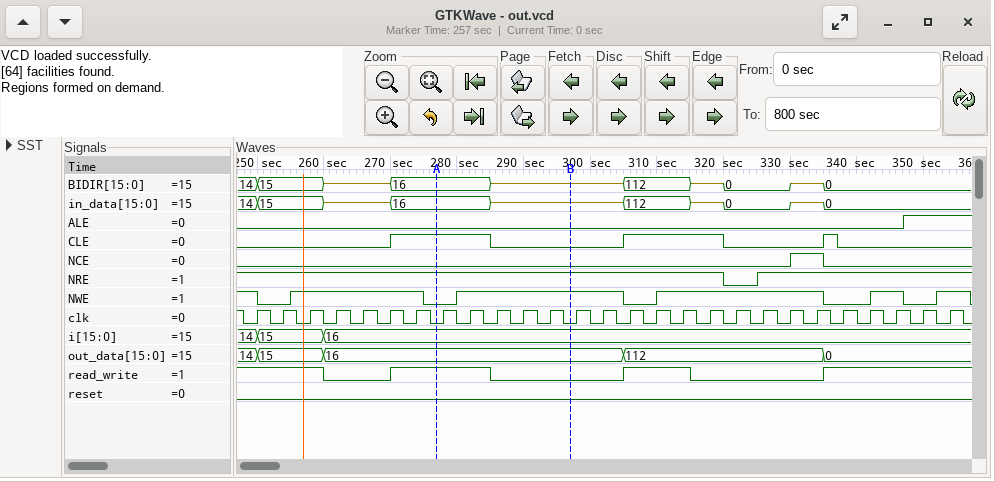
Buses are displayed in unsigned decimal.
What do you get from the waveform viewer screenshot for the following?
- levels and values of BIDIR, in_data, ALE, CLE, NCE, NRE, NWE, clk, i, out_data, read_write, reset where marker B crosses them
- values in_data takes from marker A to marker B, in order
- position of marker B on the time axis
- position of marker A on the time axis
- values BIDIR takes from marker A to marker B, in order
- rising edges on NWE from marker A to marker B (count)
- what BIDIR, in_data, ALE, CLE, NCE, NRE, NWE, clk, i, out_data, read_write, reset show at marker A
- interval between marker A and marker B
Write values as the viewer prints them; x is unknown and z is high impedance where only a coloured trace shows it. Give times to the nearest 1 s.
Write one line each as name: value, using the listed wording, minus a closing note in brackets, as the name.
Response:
levels and values of BIDIR, in_data, ALE, CLE, NCE, NRE, NWE, clk, i, out_data, read_write, reset where marker B crosses them: BIDIR=z, in_data=z, ALE=0, CLE=0, NCE=0, NRE=1, NWE=1, clk=0, i=16, out_data=16, read_write=0, reset=0
values in_data takes from marker A to marker B, in order: 16, z
position of marker B on the time axis: 297 s
position of marker A on the time axis: 277 s
values BIDIR takes from marker A to marker B, in order: 16, z
rising edges on NWE from marker A to marker B: 1
what BIDIR, in_data, ALE, CLE, NCE, NRE, NWE, clk, i, out_data, read_write, reset show at marker A: BIDIR=16, in_data=16, ALE=0, CLE=1, NCE=0, NRE=1, NWE=0, clk=0, i=16, out_data=16, read_write=1, reset=0
interval between marker A and marker B: 20 s
